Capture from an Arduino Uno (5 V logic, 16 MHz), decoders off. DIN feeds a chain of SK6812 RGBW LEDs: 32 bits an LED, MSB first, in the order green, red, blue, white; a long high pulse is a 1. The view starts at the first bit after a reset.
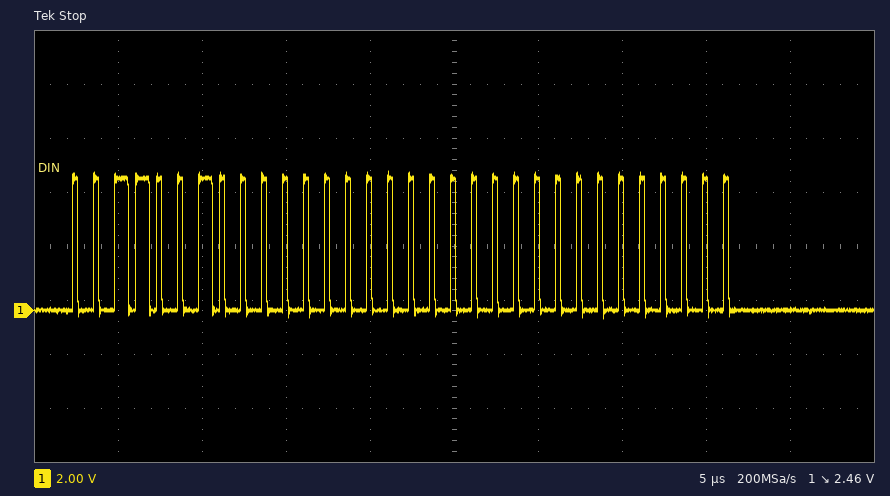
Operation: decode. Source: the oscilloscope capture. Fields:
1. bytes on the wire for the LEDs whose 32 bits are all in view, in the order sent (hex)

32 00 00 00
